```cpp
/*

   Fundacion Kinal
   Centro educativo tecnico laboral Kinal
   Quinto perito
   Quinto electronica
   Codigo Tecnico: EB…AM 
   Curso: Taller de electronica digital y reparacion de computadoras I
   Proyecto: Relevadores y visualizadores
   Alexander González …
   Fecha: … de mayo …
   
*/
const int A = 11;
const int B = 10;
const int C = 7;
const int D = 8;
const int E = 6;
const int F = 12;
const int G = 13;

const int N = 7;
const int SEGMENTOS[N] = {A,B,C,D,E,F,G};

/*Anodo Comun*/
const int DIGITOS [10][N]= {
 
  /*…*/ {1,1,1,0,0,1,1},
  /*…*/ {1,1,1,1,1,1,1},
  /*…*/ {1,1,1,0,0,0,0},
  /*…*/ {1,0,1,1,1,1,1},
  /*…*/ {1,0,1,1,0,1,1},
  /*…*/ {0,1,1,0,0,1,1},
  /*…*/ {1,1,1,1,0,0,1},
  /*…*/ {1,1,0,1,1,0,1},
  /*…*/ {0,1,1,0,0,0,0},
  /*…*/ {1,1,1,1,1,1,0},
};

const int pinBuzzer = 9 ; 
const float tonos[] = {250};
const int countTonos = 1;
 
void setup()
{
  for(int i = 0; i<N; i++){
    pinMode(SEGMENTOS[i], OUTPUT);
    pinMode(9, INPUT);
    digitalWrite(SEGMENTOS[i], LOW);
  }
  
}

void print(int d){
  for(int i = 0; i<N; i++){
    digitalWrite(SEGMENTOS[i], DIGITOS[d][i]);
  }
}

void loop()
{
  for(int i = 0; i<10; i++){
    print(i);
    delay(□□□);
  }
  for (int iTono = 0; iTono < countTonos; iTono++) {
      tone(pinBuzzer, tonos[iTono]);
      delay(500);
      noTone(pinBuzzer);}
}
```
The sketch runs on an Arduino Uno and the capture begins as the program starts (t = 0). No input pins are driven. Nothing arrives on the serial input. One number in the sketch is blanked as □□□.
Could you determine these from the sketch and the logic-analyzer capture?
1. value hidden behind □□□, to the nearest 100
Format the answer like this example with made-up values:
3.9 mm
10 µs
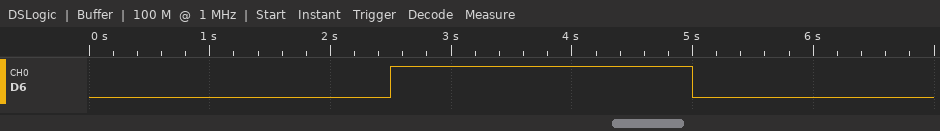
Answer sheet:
2500
